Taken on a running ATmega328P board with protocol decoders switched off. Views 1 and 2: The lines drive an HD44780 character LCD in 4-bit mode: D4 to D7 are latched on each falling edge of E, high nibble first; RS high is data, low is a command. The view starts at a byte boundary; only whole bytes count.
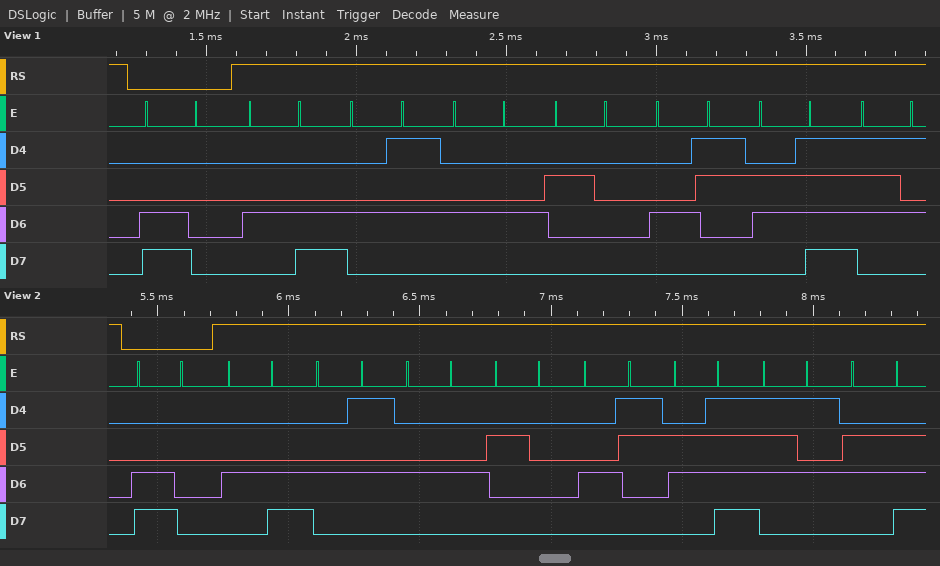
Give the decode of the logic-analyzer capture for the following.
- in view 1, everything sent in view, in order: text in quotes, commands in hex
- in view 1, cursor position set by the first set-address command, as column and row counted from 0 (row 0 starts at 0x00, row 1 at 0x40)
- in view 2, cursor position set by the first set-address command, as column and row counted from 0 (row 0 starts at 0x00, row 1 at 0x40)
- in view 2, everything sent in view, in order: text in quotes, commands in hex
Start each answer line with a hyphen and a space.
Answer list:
- 0xC0 "LED Cou"
- column 0, row 1
- column 0, row 1
- 0xC0 "LED Coun"
